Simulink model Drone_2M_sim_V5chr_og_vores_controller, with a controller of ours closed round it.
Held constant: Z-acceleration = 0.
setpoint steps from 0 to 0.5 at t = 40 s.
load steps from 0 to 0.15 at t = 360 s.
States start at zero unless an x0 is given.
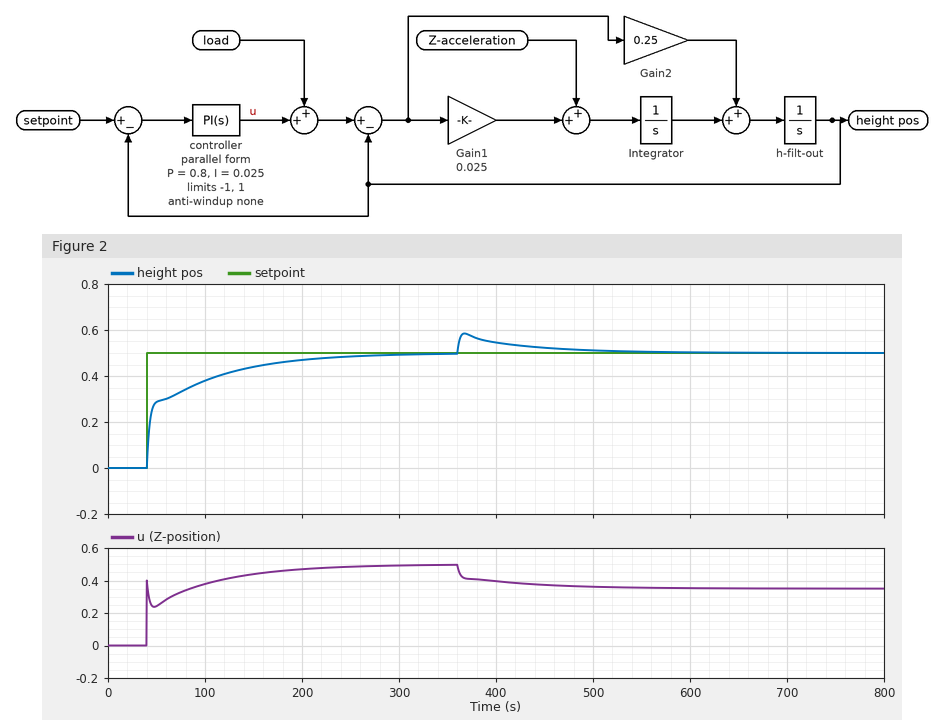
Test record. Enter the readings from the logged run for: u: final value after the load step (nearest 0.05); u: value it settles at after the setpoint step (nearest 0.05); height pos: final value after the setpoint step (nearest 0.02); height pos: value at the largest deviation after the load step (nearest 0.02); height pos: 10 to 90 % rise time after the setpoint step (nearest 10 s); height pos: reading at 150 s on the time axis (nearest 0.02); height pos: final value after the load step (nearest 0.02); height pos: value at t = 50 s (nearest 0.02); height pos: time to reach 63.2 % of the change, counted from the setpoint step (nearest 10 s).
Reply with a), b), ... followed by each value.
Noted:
a) 0.35
b) 0.50
c) 0.50
d) 0.58
e) 120 s
f) 0.44
g) 0.50
h) 0.28
i) 30 s
